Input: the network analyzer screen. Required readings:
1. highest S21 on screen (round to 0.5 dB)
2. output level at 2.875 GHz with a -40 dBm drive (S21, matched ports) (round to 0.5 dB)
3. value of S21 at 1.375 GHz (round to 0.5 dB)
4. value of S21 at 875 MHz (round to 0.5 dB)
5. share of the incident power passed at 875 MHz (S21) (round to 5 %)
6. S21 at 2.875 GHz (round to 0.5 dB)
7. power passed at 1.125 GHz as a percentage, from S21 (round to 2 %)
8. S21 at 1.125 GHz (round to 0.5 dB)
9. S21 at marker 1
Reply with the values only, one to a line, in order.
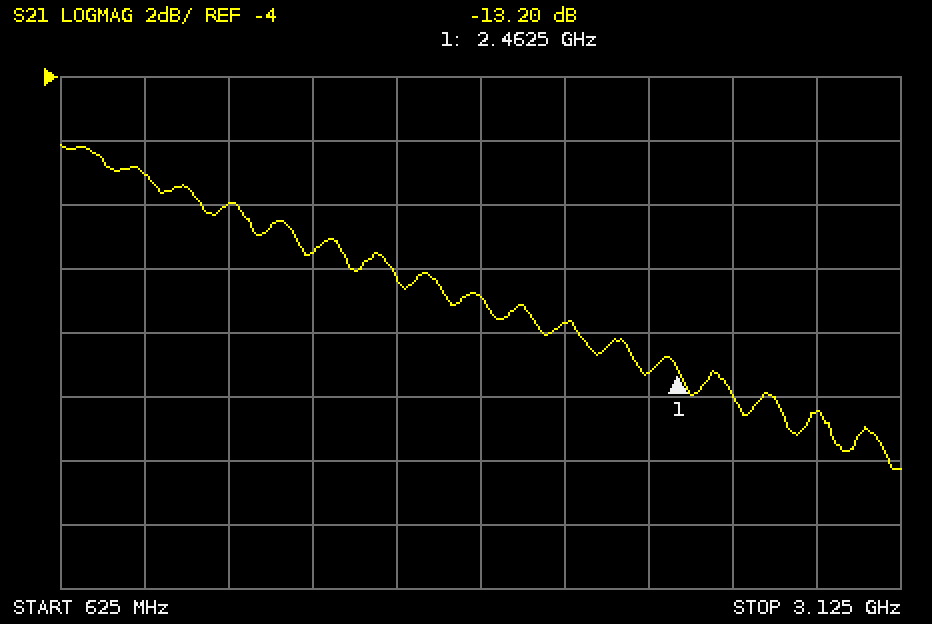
-6.0 dB
-54.5 dBm
-9.5 dB
-7.0 dB
20 %
-14.5 dB
16 %
-8.0 dB
-13.20 dB
